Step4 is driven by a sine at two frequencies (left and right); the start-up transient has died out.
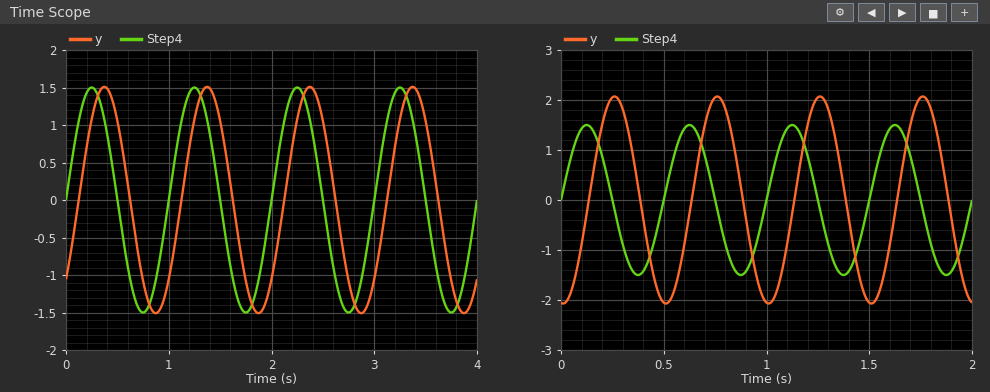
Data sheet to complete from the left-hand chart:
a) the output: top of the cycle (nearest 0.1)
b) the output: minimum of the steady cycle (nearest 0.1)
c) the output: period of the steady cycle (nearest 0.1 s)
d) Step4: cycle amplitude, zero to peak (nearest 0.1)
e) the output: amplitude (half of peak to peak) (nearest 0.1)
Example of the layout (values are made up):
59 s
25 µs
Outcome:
1.5
-1.5
1.0 s
1.5
1.5
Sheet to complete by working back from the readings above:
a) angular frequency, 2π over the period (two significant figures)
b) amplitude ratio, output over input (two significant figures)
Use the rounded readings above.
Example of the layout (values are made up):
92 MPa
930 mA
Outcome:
6.3 rad/s
1.0
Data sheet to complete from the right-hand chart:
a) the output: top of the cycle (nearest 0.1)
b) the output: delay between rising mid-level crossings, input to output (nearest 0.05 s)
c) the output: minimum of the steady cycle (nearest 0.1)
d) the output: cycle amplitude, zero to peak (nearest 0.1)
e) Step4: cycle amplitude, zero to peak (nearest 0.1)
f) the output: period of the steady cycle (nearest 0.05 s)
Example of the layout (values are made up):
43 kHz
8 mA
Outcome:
2.1
0.15 s
-2.1
2.1
1.5
0.50 s
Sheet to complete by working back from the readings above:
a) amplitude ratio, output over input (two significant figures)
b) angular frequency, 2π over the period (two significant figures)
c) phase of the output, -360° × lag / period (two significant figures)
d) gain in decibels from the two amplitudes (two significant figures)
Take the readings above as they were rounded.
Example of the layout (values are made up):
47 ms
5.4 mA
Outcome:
1.4
13 rad/s
-110°
2.9 dB
